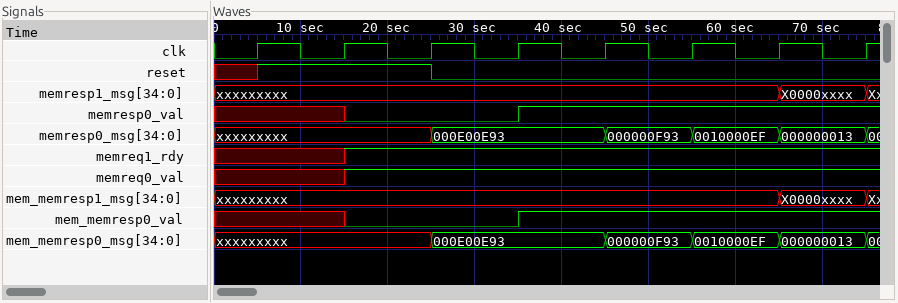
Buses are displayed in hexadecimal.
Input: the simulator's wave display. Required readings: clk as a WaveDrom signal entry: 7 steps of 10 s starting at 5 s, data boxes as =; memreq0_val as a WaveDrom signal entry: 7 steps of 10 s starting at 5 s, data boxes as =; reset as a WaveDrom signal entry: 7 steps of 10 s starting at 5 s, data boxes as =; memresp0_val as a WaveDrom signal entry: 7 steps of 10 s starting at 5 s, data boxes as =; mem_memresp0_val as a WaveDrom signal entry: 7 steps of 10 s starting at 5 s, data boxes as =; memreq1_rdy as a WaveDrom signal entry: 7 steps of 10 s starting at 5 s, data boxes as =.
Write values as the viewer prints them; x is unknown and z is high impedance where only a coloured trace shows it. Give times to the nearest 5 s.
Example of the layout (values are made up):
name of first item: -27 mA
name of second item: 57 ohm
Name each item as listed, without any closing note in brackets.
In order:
clk as a WaveDrom signal entry: 7 steps of 10 s starting at 5 s, data boxes as =: {name: 'clk', wave: 'p......'}
memreq0_val as a WaveDrom signal entry: 7 steps of 10 s starting at 5 s, data boxes as =: {name: 'memreq0_val', wave: 'x1.....'}
reset as a WaveDrom signal entry: 7 steps of 10 s starting at 5 s, data boxes as =: {name: 'reset', wave: '1.0....'}
memresp0_val as a WaveDrom signal entry: 7 steps of 10 s starting at 5 s, data boxes as =: {name: 'memresp0_val', wave: 'x0.1...'}
mem_memresp0_val as a WaveDrom signal entry: 7 steps of 10 s starting at 5 s, data boxes as =: {name: 'mem_memresp0_val', wave: 'x0.1...'}
memreq1_rdy as a WaveDrom signal entry: 7 steps of 10 s starting at 5 s, data boxes as =: {name: 'memreq1_rdy', wave: 'x1.....'}
